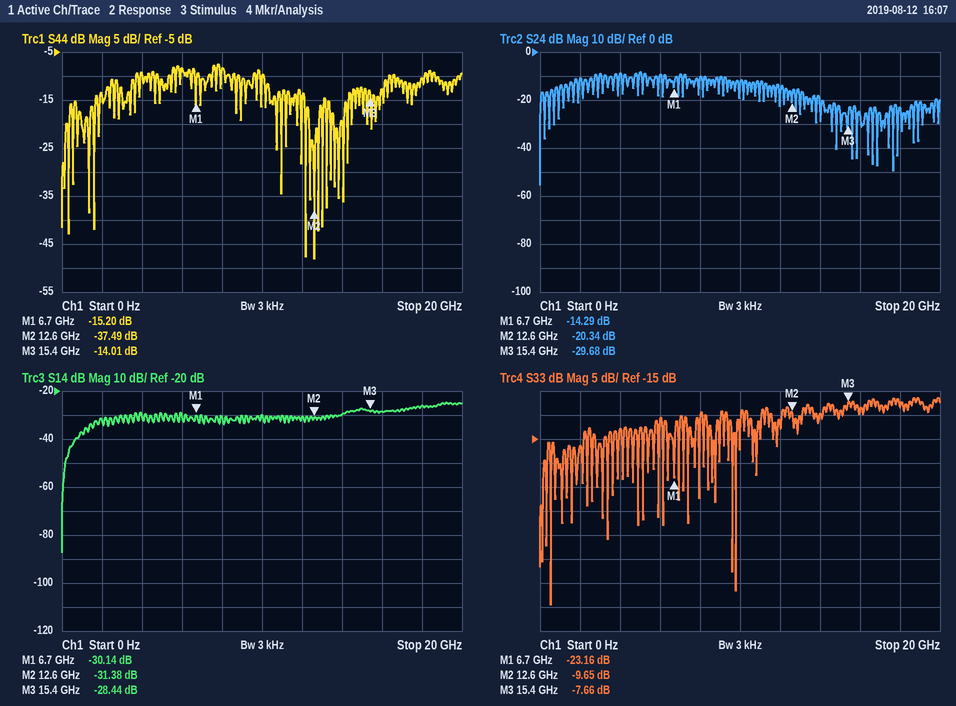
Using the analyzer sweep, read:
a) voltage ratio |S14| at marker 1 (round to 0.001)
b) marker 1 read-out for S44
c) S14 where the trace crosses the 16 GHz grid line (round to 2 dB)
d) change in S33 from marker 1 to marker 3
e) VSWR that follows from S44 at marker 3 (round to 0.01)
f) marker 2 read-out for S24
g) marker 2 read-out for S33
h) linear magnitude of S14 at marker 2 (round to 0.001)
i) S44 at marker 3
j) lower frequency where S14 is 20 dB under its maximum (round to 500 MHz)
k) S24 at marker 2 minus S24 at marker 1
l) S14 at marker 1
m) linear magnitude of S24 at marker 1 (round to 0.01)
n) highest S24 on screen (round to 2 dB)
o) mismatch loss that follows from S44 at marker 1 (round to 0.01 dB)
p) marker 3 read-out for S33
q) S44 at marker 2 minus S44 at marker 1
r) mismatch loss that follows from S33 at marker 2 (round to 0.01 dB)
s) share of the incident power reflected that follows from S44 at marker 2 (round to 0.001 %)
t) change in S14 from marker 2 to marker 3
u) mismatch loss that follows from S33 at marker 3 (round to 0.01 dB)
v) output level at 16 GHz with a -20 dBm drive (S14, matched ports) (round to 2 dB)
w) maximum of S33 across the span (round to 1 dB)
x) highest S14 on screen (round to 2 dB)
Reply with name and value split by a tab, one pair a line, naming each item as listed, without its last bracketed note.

voltage ratio |S14| at marker 1	0.031
marker 1 read-out for S44	-15.20 dB
S14 where the trace crosses the 16 GHz grid line	-28 dB
change in S33 from marker 1 to marker 3	15.50 dB
VSWR that follows from S44 at marker 3	1.50
marker 2 read-out for S24	-20.34 dB
marker 2 read-out for S33	-9.65 dB
linear magnitude of S14 at marker 2	0.027
S44 at marker 3	-14.01 dB
lower frequency where S14 is 20 dB under its maximum	500 MHz
S24 at marker 2 minus S24 at marker 1	-6.05 dB
S14 at marker 1	-30.14 dB
linear magnitude of S24 at marker 1	0.19
highest S24 on screen	-8 dB
mismatch loss that follows from S44 at marker 1	0.13 dB
marker 3 read-out for S33	-7.66 dB
S44 at marker 2 minus S44 at marker 1	-22.29 dB
mismatch loss that follows from S33 at marker 2	0.50 dB
share of the incident power reflected that follows from S44 at marker 2	0.018 %
change in S14 from marker 2 to marker 3	2.94 dB
mismatch loss that follows from S33 at marker 3	0.82 dB
output level at 16 GHz with a -20 dBm drive (S14, matched ports)	-48 dBm
maximum of S33 across the span	-6 dB
highest S14 on screen	-24 dB
